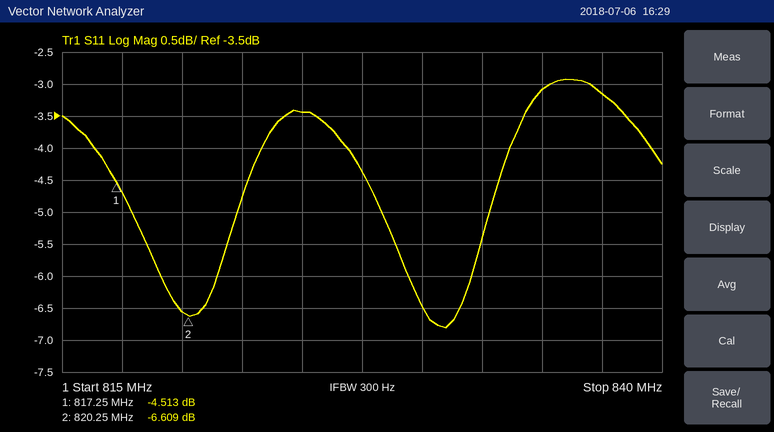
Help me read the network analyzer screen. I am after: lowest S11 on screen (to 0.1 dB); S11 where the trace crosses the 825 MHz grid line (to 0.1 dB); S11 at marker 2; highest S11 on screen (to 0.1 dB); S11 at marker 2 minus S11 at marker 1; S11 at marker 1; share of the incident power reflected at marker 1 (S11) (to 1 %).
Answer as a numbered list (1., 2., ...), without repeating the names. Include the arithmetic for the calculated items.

1. -6.8 dB
2. -3.4 dB
3. -6.609 dB
4. -2.9 dB
5. -6.609 − (-4.513) = -2.096 dB
6. -4.513 dB
7. 10^(-4.513/10) ≈ 35 %
